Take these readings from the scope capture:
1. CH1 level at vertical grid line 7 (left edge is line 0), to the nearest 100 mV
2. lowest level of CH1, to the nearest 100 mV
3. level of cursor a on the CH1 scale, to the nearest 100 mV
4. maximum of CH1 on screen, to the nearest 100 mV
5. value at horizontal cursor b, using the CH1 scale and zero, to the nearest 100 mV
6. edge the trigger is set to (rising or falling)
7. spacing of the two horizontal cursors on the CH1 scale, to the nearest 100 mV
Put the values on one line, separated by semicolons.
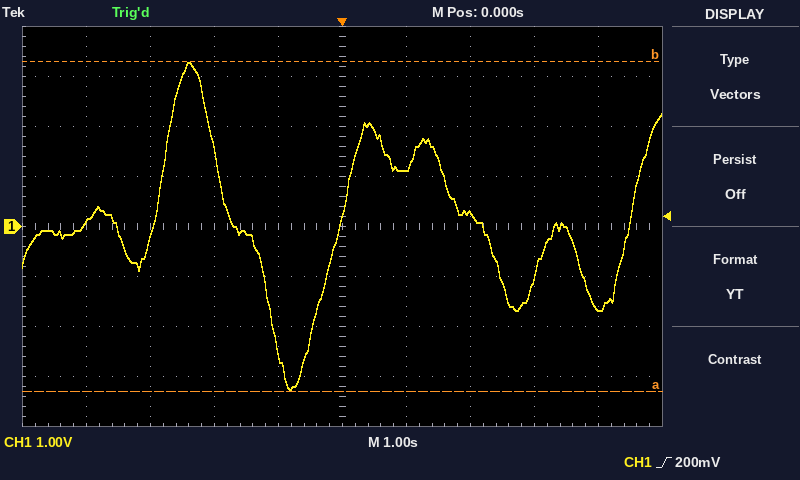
300 mV; -3.3 V; -3.3 V; 3.3 V; 3.3 V; rising; 6.6 V
